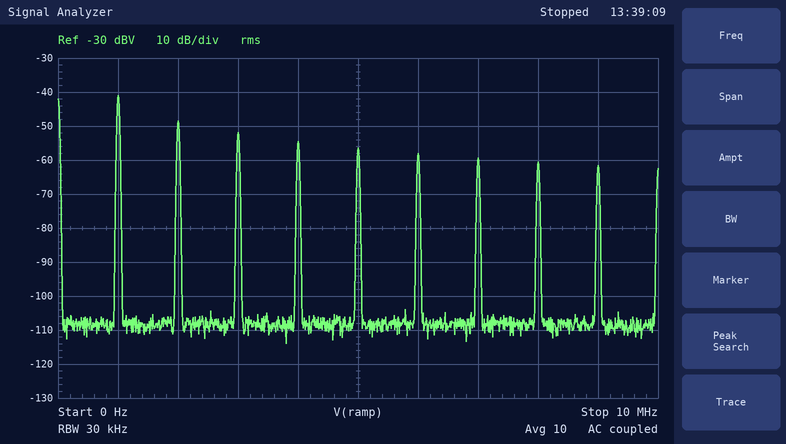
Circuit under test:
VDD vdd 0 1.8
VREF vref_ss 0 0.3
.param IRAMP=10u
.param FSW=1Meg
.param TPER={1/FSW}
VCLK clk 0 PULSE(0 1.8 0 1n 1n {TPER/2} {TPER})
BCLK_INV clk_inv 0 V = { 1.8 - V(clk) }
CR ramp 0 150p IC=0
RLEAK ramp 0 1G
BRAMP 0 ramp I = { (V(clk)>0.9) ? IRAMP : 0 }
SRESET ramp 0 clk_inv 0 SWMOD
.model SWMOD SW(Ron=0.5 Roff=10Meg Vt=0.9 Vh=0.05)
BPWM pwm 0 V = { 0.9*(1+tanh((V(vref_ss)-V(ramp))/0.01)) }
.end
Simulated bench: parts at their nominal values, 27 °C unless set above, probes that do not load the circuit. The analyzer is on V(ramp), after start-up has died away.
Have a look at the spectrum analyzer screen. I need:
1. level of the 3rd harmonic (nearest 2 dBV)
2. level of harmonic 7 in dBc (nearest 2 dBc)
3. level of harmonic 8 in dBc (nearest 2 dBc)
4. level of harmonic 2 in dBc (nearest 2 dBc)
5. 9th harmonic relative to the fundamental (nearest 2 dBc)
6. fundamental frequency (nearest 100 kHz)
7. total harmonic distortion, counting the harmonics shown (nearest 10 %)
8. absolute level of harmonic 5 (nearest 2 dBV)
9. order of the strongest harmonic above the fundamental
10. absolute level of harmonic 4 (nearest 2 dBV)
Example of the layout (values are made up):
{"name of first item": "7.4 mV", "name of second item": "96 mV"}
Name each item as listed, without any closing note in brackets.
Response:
{"level of the 3rd harmonic": "-52 dBV", "level of harmonic 7 in dBc": "-18 dBc", "level of harmonic 8 in dBc": "-20 dBc", "level of harmonic 2 in dBc": "-8 dBc", "9th harmonic relative to the fundamental": "-20 dBc", "fundamental frequency": "1.0 MHz", "total harmonic distortion, counting the harmonics shown": "60 %", "absolute level of harmonic 5": "-56 dBV", "order of the strongest harmonic above the fundamental": "2", "absolute level of harmonic 4": "-54 dBV"}
